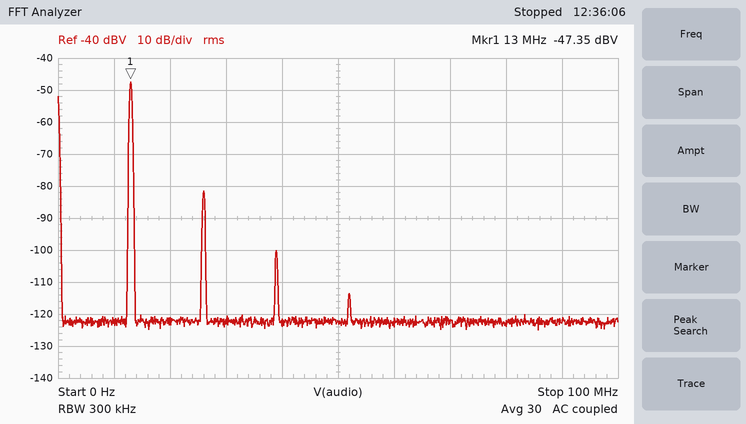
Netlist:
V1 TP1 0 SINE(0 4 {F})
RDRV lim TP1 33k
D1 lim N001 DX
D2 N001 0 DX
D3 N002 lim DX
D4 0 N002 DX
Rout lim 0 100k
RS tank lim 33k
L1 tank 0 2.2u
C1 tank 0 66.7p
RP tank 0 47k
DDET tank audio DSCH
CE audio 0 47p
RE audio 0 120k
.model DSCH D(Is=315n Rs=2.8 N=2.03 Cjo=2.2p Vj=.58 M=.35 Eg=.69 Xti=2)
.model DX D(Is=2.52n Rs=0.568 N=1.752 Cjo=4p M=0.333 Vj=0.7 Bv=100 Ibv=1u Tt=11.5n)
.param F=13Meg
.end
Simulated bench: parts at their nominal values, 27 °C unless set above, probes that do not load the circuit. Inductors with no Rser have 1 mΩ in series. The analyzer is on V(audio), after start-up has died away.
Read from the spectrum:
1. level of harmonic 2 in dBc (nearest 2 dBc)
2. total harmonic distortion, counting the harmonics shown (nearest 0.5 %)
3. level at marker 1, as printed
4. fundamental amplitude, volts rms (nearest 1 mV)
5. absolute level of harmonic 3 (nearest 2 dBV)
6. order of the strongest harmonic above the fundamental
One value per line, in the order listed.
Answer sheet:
-34 dBc
2.0 %
-47.35 dBV
4 mV
-100 dBV
2
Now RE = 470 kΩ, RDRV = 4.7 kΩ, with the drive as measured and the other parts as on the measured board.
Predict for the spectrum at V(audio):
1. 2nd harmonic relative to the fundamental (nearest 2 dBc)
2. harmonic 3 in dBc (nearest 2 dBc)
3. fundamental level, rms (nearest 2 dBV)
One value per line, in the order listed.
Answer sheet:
-26 dBc
-42 dBc
-36 dBV
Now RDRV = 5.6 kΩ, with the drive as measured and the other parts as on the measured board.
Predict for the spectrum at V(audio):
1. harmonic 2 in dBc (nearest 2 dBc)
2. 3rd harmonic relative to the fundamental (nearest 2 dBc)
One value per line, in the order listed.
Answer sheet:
-26 dBc
-38 dBc
